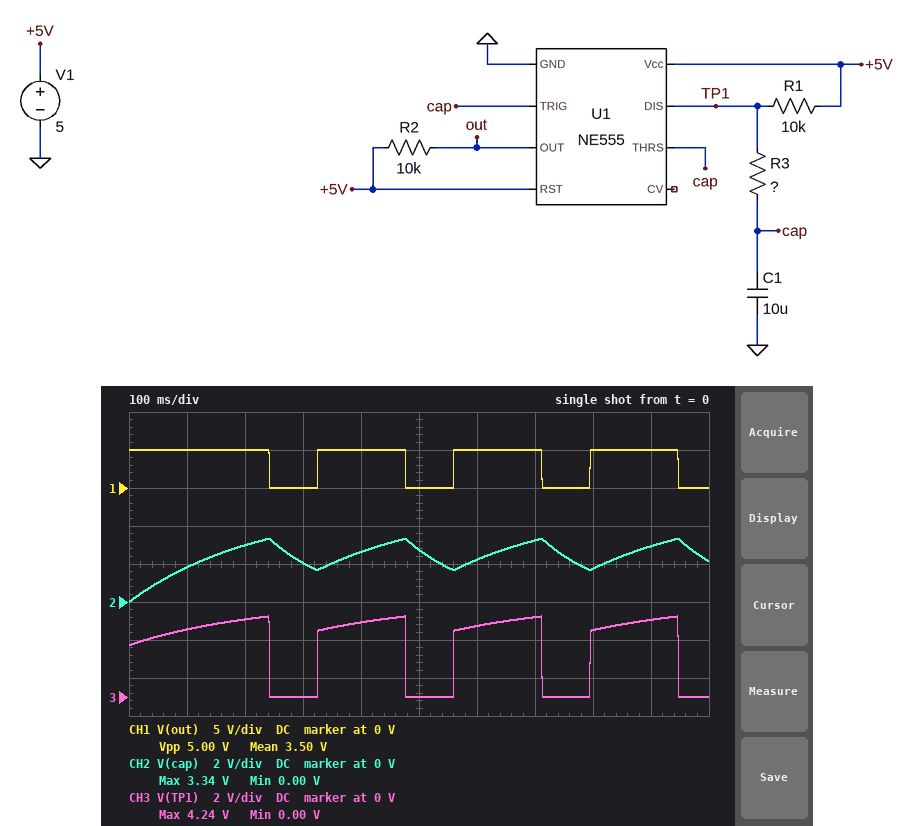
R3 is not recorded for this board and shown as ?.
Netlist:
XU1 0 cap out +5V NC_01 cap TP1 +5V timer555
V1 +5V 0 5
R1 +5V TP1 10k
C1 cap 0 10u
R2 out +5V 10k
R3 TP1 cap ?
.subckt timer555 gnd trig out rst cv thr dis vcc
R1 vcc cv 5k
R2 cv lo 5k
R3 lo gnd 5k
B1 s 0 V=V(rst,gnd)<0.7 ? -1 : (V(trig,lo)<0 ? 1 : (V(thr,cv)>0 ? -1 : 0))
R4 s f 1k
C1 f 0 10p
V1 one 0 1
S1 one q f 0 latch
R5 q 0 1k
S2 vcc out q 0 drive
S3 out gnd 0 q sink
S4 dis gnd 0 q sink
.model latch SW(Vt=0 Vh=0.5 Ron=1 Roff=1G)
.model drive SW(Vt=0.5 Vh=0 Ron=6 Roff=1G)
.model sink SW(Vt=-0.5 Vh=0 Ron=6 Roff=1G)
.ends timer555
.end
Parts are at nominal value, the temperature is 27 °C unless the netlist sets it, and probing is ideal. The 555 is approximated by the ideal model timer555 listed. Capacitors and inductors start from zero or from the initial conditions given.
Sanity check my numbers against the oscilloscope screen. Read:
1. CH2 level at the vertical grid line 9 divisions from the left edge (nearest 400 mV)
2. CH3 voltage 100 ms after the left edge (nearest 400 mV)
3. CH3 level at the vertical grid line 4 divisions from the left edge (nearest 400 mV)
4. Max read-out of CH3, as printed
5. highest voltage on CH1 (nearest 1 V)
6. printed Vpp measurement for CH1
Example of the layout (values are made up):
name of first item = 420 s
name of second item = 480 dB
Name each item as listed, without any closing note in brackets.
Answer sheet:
CH2 level at the vertical grid line 9 divisions from the left edge = 2.8 V
CH3 voltage 100 ms after the left edge = 3.6 V
CH3 level at the vertical grid line 4 divisions from the left edge = 4.0 V
Max read-out of CH3, as printed = 4.24 V
highest voltage on CH1 = 5 V
printed Vpp measurement for CH1 = 5.00 V
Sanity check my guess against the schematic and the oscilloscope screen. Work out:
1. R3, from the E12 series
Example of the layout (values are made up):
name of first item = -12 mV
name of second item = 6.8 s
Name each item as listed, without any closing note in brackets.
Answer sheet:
R3, from the E12 series = 12 kΩ
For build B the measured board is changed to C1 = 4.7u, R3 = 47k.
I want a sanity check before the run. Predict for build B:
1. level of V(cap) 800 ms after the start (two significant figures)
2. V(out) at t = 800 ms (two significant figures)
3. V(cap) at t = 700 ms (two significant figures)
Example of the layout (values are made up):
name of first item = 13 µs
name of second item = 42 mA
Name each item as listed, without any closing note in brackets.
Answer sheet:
level of V(cap) 800 ms after the start = 1.8 V
V(out) at t = 800 ms = 5.0 V
V(cap) at t = 700 ms = 2.5 V
